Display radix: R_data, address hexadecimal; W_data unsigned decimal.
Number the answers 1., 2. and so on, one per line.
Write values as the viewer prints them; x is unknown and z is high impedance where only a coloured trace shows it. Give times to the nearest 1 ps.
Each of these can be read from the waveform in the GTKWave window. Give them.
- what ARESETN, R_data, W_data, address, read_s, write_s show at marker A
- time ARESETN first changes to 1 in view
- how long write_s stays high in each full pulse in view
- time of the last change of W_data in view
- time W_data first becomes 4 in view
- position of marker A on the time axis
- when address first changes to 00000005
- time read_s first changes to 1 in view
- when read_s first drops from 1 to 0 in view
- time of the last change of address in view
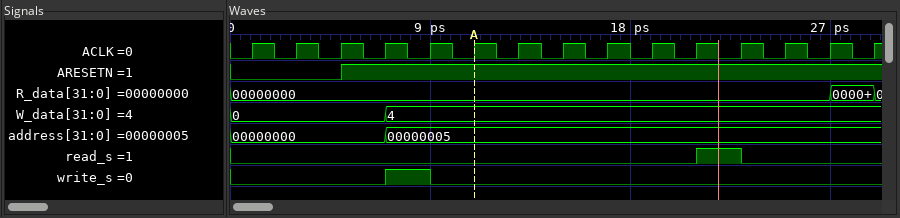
1. ARESETN=1, R_data=00000000, W_data=4, address=00000005, read_s=0, write_s=0
2. 5 ps
3. 2 ps
4. 7 ps
5. 7 ps
6. 11 ps
7. 7 ps
8. 21 ps
9. 23 ps
10. 7 ps
